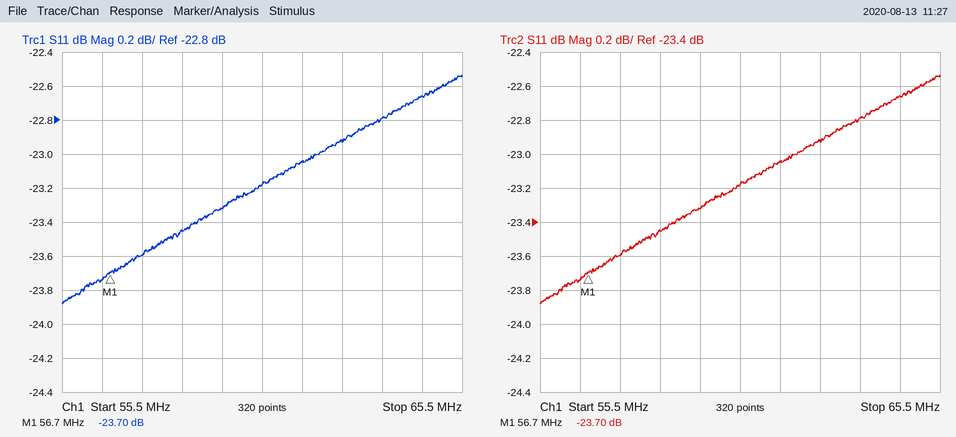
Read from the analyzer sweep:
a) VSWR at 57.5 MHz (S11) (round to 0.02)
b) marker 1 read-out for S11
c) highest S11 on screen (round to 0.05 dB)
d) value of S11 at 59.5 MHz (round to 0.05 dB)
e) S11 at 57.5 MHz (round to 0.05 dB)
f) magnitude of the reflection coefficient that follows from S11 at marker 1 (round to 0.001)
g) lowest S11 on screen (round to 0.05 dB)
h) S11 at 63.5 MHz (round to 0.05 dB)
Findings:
1.14
-23.70 dB
-22.55 dB
-23.30 dB
-23.60 dB
0.065
-23.90 dB
-22.80 dB
